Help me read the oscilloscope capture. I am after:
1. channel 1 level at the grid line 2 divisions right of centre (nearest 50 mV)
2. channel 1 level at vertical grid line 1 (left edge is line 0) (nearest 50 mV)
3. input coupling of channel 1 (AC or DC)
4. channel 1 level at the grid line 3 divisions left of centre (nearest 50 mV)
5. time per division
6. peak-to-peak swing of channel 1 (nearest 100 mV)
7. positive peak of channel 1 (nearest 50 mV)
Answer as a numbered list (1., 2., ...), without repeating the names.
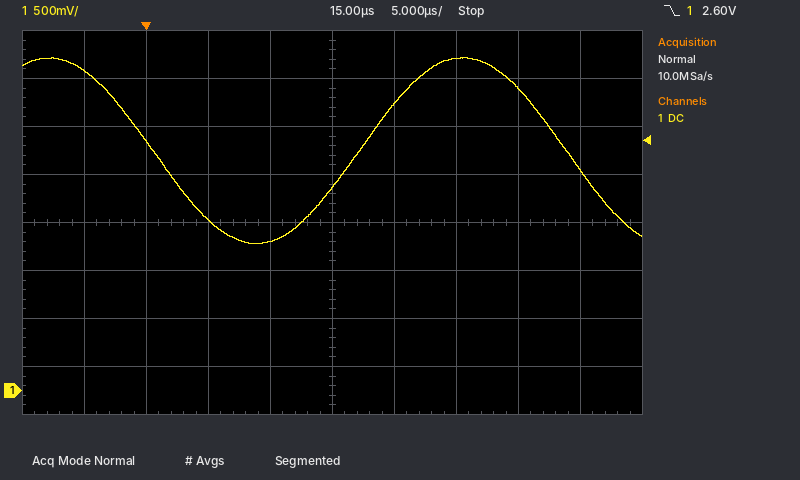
1. 3.45 V
2. 3.35 V
3. DC
4. 2.60 V
5. 5 µs
6. 1.90 V
7. 3.45 V
